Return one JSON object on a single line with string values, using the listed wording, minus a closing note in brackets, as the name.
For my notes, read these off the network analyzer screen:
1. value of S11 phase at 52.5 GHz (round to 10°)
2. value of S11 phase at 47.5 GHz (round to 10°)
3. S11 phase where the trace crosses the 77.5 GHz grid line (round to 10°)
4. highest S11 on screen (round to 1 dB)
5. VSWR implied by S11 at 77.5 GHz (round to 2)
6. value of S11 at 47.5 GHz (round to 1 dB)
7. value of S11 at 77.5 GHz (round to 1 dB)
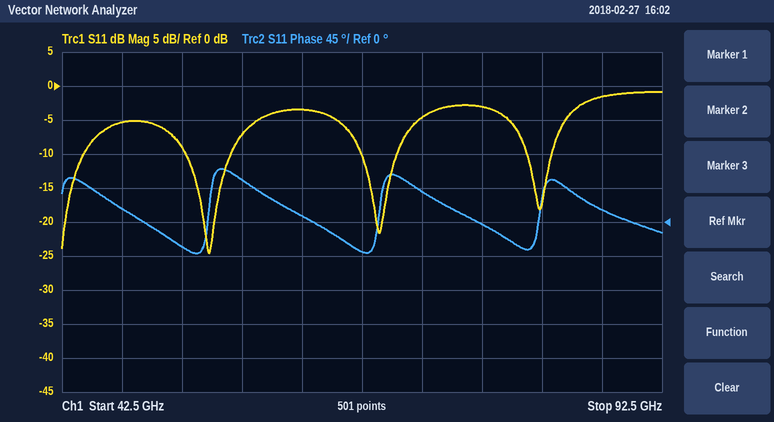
{"value of S11 phase at 52.5 GHz": "-30°", "value of S11 phase at 47.5 GHz": "20°", "S11 phase where the trace crosses the 77.5 GHz grid line": "0°", "highest S11 on screen": "-1 dB", "VSWR implied by S11 at 77.5 GHz": "6", "value of S11 at 47.5 GHz": "-5 dB", "value of S11 at 77.5 GHz": "-3 dB"}
